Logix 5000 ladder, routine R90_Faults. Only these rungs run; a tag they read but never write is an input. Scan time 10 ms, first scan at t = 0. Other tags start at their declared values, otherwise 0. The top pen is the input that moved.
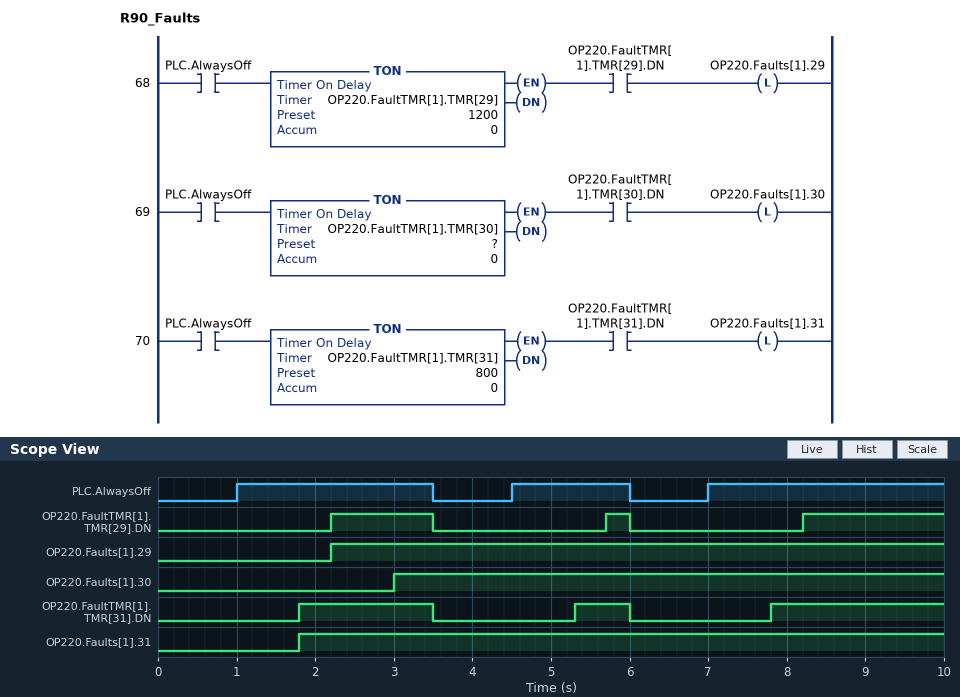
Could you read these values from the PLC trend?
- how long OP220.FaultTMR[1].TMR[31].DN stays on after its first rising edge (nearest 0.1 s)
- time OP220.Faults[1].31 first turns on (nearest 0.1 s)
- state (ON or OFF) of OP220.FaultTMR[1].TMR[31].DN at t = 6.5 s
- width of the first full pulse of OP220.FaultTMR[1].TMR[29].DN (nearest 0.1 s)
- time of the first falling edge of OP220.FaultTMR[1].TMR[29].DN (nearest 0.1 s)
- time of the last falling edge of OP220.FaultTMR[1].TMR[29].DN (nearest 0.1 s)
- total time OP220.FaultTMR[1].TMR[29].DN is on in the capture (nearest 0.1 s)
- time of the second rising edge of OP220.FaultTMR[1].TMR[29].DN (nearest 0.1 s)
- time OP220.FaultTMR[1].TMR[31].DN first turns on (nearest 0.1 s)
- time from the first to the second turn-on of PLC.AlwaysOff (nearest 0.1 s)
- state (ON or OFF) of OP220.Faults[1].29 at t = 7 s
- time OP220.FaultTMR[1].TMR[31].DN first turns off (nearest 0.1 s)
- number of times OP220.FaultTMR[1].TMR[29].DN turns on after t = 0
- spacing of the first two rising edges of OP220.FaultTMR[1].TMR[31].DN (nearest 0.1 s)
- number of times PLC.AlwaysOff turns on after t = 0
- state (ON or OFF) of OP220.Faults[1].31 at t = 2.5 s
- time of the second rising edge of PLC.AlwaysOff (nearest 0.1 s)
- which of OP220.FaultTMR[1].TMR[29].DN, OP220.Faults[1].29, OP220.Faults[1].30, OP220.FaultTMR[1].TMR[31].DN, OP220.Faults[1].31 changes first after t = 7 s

1.7 s
1.8 s
OFF
1.3 s
3.5 s
6.0 s
3.4 s
5.7 s
1.8 s
3.5 s
ON
3.5 s
3
3.5 s
3
ON
4.5 s
OP220.FaultTMR[1].TMR[31].DN
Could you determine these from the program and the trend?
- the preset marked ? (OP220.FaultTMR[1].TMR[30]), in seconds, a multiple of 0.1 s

2.0 s
